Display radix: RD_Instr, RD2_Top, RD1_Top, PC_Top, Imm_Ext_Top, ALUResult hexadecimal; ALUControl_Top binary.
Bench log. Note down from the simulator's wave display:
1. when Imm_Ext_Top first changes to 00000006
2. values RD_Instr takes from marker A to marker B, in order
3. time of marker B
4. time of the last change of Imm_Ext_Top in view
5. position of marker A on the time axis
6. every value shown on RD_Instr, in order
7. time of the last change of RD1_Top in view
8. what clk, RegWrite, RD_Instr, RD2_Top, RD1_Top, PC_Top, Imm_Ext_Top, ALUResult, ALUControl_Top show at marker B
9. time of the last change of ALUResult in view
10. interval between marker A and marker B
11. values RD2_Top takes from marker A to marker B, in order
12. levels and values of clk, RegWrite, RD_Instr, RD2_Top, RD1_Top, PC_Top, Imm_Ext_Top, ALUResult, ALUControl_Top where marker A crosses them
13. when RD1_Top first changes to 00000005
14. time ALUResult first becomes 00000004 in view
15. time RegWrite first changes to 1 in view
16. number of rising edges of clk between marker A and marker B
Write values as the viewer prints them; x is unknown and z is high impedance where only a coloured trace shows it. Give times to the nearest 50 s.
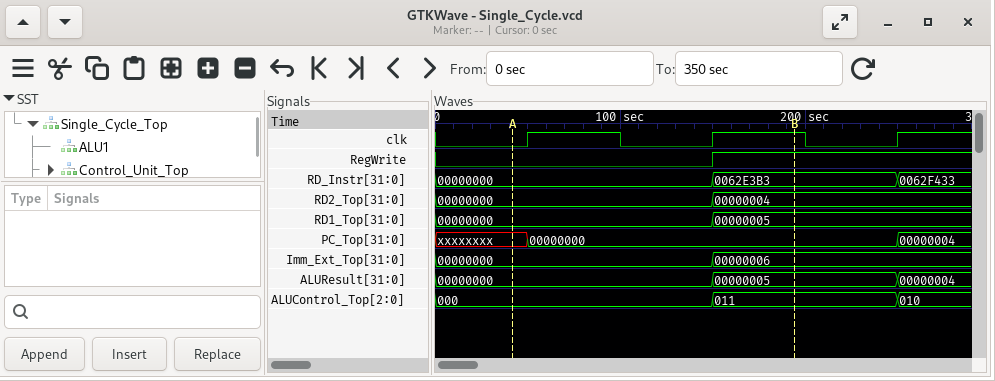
150 s
00000000, 0062E3B3
200 s
150 s
50 s
00000000, 0062E3B3, 0062F433
150 s
clk=1, RegWrite=1, RD_Instr=0062E3B3, RD2_Top=00000004, RD1_Top=00000005, PC_Top=00000000, Imm_Ext_Top=00000006, ALUResult=00000005, ALUControl_Top=011
250 s
150 s
00000000, 00000004
clk=0, RegWrite=0, RD_Instr=00000000, RD2_Top=00000000, RD1_Top=00000000, PC_Top=xxxxxxxx, Imm_Ext_Top=00000000, ALUResult=00000000, ALUControl_Top=000
150 s
250 s
150 s
2
